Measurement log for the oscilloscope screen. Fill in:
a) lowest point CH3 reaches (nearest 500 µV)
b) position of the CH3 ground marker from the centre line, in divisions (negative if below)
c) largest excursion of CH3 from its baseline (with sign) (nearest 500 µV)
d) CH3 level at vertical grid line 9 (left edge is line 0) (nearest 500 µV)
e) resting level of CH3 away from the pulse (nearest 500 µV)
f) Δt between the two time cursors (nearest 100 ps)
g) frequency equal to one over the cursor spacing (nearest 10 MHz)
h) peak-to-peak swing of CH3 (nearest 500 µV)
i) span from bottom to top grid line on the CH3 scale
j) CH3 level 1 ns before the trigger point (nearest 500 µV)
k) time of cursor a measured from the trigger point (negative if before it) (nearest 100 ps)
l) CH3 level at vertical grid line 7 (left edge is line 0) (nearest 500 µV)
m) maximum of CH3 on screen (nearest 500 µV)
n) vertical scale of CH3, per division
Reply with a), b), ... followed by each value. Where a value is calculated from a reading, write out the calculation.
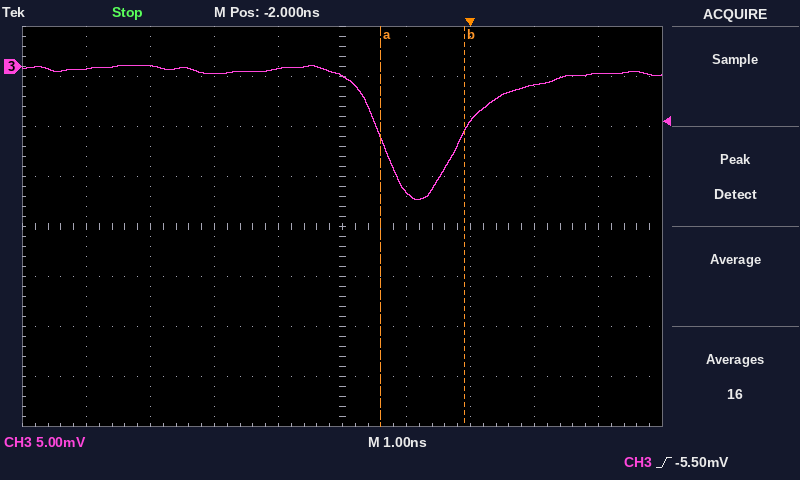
a) -13.5 mV
b) +3.2 div
c) -13.5 mV − (-500 µV) = -13.0 mV
d) -500 µV
e) -500 µV
f) 1.3 ns
g) 1 / 1.3 ns ≈ 770 MHz
h) 0.0 mV − (-13.5 mV) = 13.5 mV
i) 40 mV
j) -12.5 mV
k) -1.4 ns
l) -5.5 mV
m) 0.0 mV
n) 5 mV
